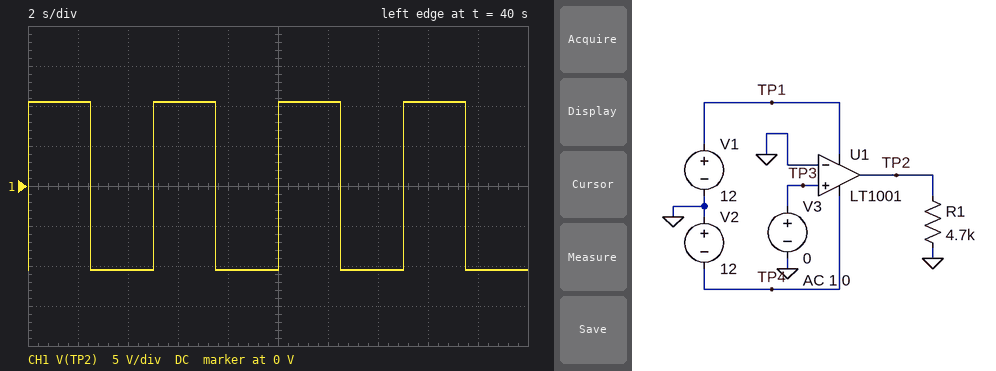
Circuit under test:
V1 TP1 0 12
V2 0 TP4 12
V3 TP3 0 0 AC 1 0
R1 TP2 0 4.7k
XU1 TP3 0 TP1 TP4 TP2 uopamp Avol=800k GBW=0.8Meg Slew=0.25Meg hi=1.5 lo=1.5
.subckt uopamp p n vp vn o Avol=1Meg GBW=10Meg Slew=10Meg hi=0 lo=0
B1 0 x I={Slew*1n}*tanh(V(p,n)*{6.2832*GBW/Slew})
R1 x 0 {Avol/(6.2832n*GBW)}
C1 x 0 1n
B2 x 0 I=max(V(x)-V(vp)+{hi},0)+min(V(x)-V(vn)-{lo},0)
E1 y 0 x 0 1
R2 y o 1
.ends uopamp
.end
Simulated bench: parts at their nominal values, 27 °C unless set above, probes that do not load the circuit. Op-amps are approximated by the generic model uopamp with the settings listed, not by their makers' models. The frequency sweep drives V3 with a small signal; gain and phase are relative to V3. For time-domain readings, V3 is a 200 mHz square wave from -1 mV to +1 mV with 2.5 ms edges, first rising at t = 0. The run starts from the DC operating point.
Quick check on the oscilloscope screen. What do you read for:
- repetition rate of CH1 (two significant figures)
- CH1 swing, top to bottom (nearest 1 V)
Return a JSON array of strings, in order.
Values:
["200 mHz", "21 V"]
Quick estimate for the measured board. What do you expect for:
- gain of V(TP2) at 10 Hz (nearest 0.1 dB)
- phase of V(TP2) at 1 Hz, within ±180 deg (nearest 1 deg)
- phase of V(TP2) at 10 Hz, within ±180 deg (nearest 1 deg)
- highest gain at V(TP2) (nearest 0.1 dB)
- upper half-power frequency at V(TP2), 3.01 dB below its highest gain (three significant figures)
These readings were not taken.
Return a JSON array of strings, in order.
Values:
["98.0 dB", "-45 deg", "-84 deg", "118.1 dB", "1.00 Hz"]
